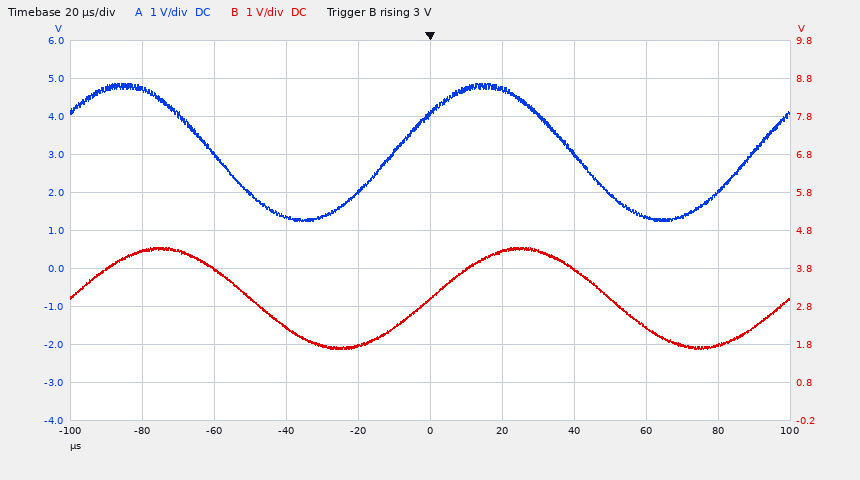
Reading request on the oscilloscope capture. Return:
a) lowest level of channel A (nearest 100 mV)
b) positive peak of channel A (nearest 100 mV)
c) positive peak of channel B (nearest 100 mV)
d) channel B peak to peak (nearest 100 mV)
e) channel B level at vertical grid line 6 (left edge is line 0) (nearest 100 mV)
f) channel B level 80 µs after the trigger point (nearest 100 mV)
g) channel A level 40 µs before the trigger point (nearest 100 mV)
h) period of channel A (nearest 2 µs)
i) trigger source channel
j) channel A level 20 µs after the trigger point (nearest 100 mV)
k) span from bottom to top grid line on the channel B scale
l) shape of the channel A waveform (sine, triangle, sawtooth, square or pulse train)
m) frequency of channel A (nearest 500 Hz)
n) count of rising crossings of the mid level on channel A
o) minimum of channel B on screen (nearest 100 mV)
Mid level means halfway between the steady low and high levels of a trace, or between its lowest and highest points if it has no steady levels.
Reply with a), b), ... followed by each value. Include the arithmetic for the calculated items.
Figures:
a) 1.2 V
b) 4.9 V
c) 4.4 V
d) 4.4 V − (1.7 V) = 2.7 V
e) 4.2 V
f) 1.8 V
g) 1.3 V
h) 100 µs
i) channel B
j) 4.7 V
k) 10 V
l) sine
m) 1 / 100 µs ≈ 10.0 kHz
n) 2
o) 1.7 V
